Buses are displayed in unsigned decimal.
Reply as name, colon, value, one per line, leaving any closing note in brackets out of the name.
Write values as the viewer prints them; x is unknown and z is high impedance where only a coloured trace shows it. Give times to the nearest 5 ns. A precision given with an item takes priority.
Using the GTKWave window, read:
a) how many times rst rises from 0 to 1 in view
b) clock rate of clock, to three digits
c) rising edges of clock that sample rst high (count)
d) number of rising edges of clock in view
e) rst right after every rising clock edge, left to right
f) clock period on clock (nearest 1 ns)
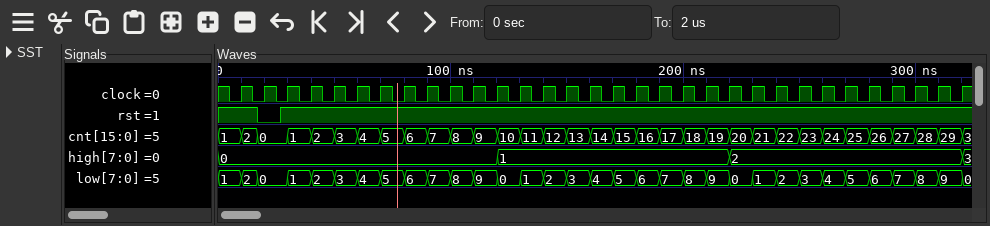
how many times rst rises from 0 to 1 in view: 1
clock rate of clock, to three digits: 100 MHz
rising edges of clock that sample rst high: 31
number of rising edges of clock in view: 32
rst right after every rising clock edge, left to right: 1 0 1 1 1 1 1 1 1 1 1 1 1 1 1 1 1 1 1 1 1 1 1 1 1 1 1 1 1 1 1 1
clock period on clock: 10 ns
